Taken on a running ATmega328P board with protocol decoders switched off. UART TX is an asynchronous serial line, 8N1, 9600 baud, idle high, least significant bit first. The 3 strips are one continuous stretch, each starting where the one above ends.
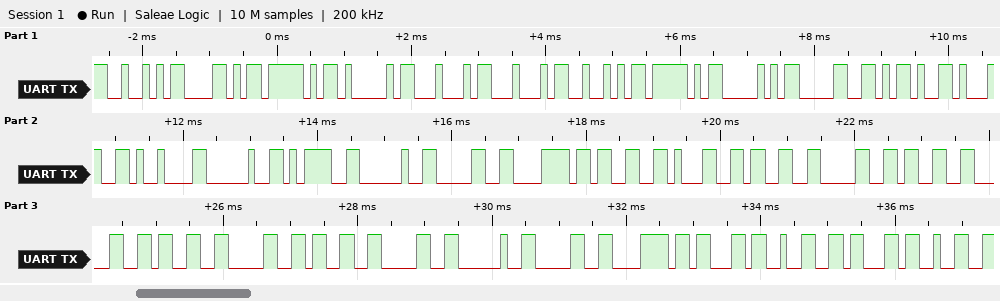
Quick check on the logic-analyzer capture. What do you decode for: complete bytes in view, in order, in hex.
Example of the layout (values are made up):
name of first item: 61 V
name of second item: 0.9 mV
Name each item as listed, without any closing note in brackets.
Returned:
complete bytes in view, in order, in hex: 52 58 5F 41 44 44 52 5F 50 30 2D 31 09 20 3D 20 30 78 33 31 33 30 33 30 33 30 33 30 20 30 78 63 32 63 32
